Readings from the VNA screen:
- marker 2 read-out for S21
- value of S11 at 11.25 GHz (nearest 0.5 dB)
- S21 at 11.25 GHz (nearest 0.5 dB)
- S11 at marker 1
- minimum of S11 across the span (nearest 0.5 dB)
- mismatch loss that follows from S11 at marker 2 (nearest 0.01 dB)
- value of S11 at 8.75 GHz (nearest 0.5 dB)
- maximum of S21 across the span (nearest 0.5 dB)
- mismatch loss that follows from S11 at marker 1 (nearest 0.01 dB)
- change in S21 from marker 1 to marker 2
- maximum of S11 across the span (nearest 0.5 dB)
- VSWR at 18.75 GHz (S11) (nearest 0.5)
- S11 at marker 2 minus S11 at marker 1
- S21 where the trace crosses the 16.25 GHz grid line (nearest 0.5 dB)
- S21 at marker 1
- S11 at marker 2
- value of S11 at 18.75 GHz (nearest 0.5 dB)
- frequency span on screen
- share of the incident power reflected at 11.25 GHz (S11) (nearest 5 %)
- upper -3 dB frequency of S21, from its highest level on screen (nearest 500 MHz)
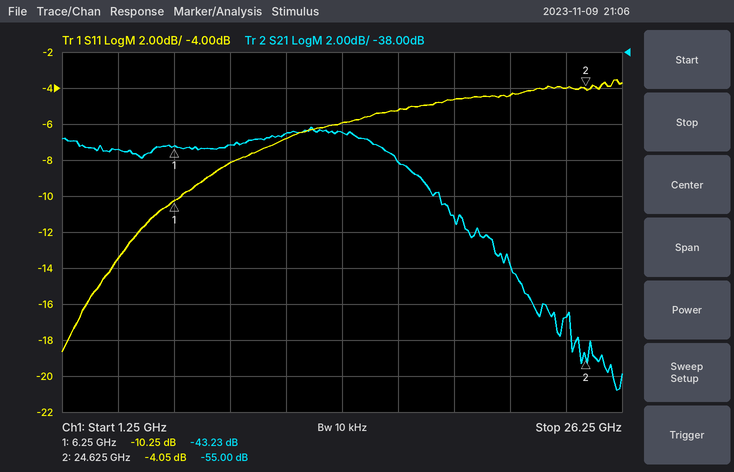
-55.00 dB
-7.0 dB
-42.5 dB
-10.25 dB
-18.5 dB
2.17 dB
-8.0 dB
-42.0 dB
0.43 dB
-11.77 dB
-3.5 dB
4.0
6.20 dB
-44.0 dB
-43.23 dB
-4.05 dB
-4.5 dB
25 GHz
20 %
17.5 GHz
